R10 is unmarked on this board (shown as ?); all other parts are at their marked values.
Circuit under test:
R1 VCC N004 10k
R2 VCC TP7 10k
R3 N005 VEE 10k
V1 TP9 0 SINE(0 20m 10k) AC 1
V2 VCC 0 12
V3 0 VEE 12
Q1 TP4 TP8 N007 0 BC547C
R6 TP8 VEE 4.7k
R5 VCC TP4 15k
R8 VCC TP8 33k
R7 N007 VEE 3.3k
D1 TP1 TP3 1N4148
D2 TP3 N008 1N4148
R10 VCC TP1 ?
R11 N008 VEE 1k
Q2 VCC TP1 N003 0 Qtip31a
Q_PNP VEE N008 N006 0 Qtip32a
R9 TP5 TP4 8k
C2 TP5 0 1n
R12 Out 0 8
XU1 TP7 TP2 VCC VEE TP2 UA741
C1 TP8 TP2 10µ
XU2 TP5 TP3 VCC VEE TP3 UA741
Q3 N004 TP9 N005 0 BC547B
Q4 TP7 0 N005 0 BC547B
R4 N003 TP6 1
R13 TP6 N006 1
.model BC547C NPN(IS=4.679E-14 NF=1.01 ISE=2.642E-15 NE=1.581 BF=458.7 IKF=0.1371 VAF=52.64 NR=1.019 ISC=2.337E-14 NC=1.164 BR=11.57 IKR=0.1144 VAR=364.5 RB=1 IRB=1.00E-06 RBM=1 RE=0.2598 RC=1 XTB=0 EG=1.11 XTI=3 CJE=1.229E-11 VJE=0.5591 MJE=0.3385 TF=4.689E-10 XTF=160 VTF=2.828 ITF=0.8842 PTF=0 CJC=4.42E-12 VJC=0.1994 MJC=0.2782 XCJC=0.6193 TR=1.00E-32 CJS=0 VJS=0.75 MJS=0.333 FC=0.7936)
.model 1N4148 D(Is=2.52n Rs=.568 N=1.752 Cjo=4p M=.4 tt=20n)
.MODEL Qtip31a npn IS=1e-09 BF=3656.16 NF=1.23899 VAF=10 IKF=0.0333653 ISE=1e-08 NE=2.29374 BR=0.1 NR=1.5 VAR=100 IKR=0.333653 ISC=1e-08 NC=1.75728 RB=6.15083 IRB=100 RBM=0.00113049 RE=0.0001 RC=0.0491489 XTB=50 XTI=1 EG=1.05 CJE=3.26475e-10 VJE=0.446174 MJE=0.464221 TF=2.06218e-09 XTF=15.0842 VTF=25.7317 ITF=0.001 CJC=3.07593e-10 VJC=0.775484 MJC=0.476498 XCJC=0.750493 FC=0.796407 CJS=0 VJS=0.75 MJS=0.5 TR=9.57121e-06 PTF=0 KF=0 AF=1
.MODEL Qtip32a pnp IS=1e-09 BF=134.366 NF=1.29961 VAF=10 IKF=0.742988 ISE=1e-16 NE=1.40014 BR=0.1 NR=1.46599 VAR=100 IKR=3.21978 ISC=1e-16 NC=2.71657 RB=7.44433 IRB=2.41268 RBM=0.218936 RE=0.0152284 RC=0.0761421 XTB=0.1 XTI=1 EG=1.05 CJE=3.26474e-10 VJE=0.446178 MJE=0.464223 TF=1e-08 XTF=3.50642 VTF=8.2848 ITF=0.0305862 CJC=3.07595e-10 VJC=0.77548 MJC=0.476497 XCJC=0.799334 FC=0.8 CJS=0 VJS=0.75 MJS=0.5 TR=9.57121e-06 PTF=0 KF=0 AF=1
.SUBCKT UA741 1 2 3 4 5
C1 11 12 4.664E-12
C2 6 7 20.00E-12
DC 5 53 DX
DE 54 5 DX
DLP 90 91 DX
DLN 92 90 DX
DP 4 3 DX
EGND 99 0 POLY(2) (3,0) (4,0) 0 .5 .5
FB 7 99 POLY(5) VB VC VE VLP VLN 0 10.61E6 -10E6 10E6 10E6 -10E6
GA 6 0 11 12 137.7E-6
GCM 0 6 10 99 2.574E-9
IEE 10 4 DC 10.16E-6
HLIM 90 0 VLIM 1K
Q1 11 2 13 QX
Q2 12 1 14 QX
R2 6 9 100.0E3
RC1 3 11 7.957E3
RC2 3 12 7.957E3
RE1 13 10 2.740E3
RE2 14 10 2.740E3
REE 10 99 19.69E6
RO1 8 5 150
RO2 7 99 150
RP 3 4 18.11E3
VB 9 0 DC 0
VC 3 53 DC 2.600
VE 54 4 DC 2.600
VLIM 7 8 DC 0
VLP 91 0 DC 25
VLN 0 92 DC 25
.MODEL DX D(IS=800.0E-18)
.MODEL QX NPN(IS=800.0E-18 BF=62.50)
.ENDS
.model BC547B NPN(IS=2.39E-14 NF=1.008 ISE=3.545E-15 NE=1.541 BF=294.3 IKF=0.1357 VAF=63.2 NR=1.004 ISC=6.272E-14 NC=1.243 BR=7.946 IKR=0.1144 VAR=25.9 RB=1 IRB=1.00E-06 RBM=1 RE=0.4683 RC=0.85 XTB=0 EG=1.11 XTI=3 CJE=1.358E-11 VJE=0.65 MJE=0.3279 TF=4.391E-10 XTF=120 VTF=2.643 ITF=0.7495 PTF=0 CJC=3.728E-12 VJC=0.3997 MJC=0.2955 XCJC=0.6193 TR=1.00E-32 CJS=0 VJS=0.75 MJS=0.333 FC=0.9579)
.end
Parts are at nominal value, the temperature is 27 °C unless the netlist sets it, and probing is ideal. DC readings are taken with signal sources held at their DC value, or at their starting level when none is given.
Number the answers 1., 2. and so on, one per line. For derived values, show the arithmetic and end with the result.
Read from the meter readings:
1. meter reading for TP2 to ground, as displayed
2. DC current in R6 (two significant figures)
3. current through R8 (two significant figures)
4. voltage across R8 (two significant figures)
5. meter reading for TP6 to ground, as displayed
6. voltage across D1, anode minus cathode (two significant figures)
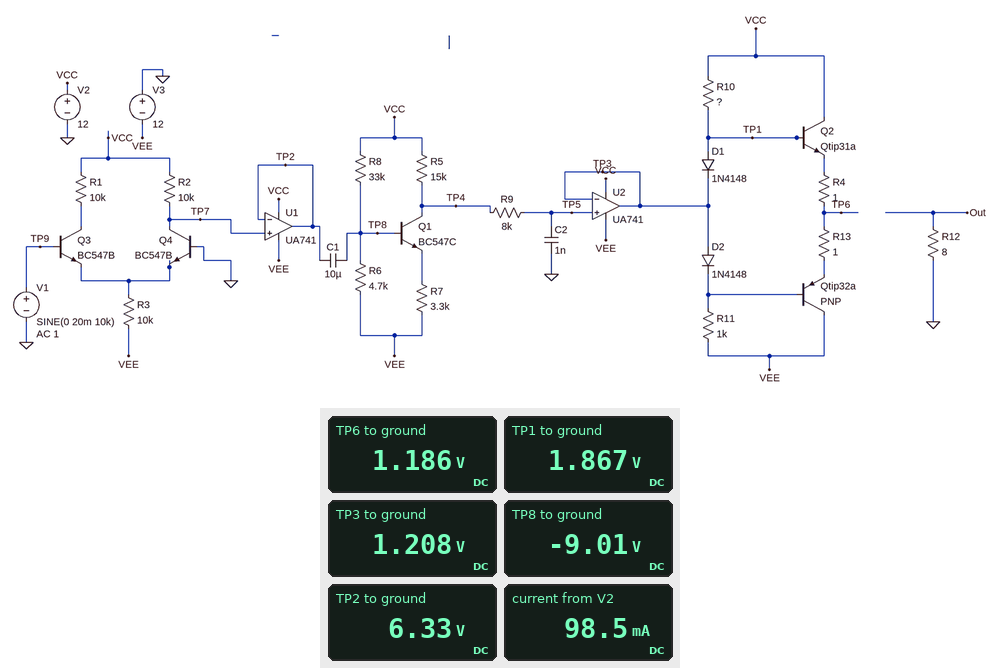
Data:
1. 6.33 V
2. (-9.01 V - (-12 V)) / 4.7 kΩ = 640 µA
3. (12 V - (-9.01 V)) / 33 kΩ = 640 µA
4. 12 V - (-9.01 V) = 21 V
5. 1.186 V
6. 1.867 V - 1.208 V = 660 mV
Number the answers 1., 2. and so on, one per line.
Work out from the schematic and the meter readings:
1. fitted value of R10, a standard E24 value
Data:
1. 2 kΩ
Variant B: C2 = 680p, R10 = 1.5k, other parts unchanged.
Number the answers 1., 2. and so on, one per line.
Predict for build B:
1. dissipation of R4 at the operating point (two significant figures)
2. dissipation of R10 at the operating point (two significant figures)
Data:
1. 8.7 mW
2. 68 mW
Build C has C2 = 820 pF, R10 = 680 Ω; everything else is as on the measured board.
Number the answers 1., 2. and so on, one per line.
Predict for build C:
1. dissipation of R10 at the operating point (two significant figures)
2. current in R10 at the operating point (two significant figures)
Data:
1. 150 mW
2. 15 mA
